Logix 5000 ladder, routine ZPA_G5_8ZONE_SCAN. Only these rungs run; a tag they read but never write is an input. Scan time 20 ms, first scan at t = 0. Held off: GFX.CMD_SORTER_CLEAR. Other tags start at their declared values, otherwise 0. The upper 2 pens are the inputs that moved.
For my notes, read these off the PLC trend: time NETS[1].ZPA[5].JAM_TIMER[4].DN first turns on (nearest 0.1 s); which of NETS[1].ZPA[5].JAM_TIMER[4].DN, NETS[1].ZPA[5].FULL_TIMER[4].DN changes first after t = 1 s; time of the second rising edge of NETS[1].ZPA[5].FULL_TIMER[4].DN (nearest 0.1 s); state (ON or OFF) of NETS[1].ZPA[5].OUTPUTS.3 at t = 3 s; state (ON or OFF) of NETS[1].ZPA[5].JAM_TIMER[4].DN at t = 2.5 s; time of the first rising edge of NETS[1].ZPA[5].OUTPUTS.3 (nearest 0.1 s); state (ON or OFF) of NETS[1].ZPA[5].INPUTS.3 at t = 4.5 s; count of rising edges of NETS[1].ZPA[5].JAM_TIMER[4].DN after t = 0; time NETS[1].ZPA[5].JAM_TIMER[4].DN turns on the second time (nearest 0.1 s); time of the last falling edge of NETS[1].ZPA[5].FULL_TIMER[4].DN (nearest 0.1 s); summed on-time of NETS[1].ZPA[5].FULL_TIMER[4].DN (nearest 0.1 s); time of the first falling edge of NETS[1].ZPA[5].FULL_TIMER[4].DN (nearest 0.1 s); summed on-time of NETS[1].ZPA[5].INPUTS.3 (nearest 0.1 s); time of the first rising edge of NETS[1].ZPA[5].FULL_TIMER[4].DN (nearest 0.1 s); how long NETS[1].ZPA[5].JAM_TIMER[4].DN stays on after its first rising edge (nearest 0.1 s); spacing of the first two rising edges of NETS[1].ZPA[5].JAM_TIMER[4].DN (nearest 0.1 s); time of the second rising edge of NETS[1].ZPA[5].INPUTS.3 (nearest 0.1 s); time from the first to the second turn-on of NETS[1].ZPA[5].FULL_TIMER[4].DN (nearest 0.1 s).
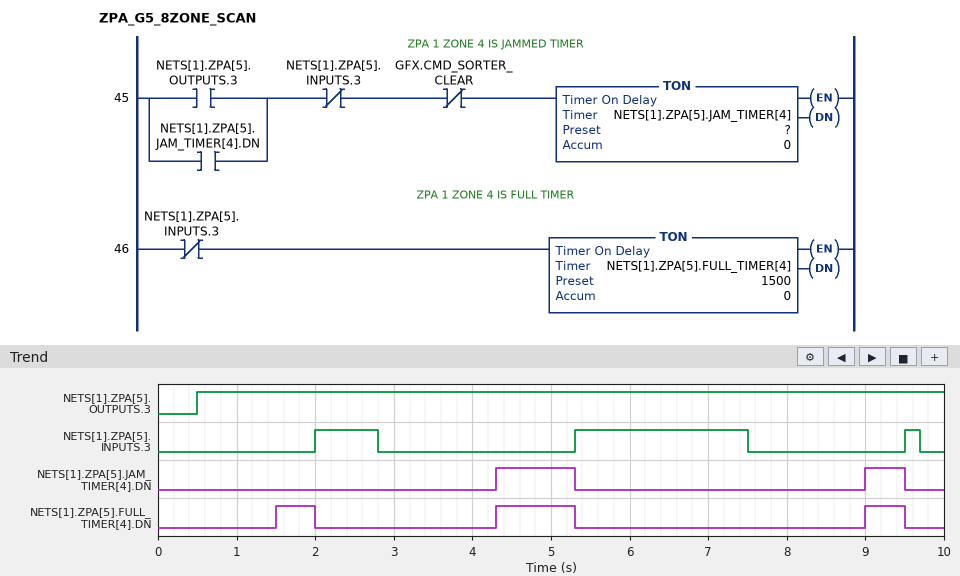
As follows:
4.3 s
NETS[1].ZPA[5].FULL_TIMER[4].DN
4.3 s
ON
OFF
0.5 s
OFF
2
9.0 s
9.5 s
2.0 s
2.0 s
3.2 s
1.5 s
1.0 s
4.7 s
5.3 s
2.8 s
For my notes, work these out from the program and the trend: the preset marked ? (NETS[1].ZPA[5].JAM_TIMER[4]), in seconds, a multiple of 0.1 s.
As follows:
1.5 s
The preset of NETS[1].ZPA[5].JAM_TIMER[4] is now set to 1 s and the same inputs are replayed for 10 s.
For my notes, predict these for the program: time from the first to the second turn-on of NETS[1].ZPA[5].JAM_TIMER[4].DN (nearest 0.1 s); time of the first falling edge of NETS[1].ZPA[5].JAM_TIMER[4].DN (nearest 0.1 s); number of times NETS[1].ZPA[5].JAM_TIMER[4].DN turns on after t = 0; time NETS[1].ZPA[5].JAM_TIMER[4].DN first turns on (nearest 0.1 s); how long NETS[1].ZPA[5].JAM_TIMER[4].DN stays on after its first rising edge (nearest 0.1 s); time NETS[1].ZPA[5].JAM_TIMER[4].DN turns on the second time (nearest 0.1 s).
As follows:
2.3 s
2.0 s
3
1.5 s
0.5 s
3.8 s
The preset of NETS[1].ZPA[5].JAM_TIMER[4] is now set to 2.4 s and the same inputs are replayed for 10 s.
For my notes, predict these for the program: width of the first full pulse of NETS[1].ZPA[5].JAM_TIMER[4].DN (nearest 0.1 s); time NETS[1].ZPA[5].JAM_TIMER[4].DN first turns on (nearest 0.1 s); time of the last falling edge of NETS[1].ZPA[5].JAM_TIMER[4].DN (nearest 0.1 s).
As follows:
0.1 s
5.2 s
5.3 s
